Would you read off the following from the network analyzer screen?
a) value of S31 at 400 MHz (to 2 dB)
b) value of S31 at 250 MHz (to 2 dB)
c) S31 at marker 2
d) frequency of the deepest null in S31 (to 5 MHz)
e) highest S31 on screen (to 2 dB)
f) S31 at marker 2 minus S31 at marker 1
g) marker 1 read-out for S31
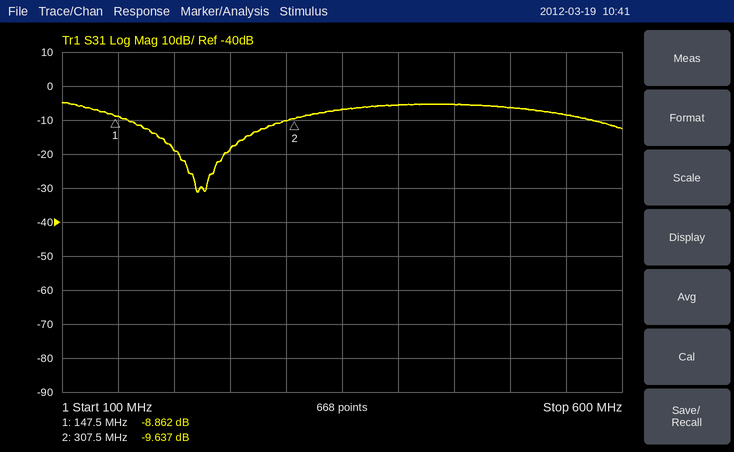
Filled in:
-6 dB
-18 dB
-9.637 dB
220 MHz
-4 dB
-0.775 dB
-8.862 dB
